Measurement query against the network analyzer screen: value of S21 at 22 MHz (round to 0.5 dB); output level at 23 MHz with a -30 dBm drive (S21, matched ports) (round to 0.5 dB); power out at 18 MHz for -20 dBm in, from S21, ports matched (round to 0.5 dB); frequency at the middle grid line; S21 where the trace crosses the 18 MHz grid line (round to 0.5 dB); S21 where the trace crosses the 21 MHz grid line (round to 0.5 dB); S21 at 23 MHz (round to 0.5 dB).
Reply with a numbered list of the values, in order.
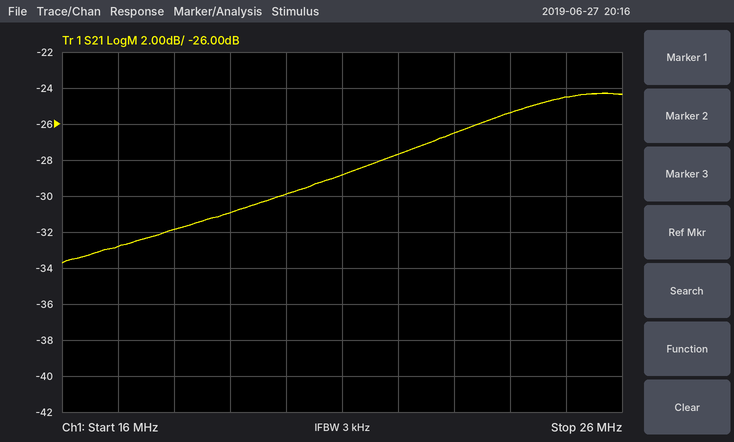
1. -27.5 dB
2. -56.5 dBm
3. -52.0 dBm
4. 21 MHz
5. -32.0 dB
6. -29.0 dB
7. -26.5 dB
